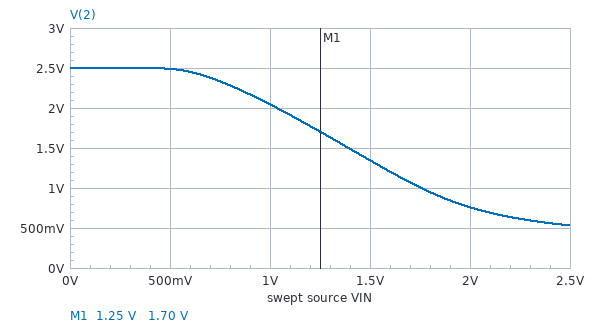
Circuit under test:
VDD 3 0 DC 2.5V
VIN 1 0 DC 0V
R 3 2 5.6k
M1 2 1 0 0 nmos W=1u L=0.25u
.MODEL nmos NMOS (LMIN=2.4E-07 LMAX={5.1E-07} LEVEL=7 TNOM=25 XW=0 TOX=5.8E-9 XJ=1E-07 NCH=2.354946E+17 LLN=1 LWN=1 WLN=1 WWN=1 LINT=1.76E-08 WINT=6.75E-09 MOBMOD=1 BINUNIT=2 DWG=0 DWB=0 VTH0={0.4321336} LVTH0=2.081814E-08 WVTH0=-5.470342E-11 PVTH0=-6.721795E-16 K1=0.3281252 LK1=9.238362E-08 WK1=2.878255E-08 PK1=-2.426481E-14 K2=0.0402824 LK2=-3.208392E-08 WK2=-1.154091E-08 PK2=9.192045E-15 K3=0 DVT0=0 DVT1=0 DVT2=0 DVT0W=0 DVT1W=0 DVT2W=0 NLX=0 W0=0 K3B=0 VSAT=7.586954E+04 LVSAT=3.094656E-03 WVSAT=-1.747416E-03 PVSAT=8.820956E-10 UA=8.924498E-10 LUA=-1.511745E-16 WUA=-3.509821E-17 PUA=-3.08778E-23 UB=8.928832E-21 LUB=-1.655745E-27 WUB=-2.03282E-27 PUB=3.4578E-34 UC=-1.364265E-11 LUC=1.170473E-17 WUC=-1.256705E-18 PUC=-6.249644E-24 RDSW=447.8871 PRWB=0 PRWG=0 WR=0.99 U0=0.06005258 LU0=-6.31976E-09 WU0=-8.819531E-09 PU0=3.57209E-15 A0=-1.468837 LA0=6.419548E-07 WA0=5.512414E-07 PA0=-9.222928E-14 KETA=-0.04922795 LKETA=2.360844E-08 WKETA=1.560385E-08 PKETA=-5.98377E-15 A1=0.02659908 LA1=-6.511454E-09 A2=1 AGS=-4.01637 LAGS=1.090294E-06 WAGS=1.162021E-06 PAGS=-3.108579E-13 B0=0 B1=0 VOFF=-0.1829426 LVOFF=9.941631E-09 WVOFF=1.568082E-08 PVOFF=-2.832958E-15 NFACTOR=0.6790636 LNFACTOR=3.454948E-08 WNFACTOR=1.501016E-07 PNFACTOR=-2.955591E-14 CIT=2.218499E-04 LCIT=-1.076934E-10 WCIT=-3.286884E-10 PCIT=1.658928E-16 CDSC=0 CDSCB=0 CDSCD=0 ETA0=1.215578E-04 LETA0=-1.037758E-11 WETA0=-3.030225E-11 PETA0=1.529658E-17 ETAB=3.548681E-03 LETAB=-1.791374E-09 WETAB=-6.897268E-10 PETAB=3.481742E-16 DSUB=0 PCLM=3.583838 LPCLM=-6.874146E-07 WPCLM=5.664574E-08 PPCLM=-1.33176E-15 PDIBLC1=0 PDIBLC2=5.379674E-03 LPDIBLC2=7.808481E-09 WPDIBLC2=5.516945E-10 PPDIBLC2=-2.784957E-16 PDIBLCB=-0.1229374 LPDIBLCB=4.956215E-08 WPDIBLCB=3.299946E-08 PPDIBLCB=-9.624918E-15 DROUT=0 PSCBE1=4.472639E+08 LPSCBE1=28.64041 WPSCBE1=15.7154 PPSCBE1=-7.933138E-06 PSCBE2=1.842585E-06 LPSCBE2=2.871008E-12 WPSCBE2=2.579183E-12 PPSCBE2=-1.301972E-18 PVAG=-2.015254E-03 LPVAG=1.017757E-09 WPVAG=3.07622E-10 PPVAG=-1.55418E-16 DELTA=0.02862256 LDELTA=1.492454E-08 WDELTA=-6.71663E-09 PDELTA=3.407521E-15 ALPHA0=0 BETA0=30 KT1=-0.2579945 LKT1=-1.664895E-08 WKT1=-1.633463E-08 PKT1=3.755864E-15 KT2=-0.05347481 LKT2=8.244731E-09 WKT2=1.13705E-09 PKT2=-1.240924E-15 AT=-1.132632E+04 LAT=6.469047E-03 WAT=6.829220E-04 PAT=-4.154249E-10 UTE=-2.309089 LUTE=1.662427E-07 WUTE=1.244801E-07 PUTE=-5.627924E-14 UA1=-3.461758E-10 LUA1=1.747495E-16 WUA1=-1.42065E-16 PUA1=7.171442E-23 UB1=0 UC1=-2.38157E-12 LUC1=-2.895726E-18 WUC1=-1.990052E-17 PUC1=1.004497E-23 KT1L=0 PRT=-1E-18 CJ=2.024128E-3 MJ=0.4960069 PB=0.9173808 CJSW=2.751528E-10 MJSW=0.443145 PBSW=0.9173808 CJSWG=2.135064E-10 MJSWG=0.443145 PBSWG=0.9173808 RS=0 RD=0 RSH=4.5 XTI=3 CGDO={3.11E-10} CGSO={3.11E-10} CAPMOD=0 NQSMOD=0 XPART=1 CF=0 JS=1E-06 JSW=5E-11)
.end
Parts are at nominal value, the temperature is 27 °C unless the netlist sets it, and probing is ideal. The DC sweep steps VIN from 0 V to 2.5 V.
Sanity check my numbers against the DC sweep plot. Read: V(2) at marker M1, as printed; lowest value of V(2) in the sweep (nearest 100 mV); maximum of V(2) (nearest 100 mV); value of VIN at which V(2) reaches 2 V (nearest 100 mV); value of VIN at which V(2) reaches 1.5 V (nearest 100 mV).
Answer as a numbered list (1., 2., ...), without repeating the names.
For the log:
1. 1.70 V
2. 500 mV
3. 2.5 V
4. 1.0 V
5. 1.4 V
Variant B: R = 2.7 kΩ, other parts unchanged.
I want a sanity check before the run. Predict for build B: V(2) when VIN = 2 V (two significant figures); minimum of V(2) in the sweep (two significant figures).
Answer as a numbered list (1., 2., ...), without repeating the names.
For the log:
1. 1.5 V
2. 1.2 V
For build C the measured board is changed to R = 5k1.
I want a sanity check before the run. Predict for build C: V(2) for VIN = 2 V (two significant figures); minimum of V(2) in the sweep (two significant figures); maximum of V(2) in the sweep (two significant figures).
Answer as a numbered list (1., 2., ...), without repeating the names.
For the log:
1. 850 mV
2. 590 mV
3. 2.5 V
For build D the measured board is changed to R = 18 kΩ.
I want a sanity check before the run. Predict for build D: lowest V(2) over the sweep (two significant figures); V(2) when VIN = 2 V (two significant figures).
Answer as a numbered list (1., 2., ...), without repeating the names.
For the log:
1. 150 mV
2. 190 mV
